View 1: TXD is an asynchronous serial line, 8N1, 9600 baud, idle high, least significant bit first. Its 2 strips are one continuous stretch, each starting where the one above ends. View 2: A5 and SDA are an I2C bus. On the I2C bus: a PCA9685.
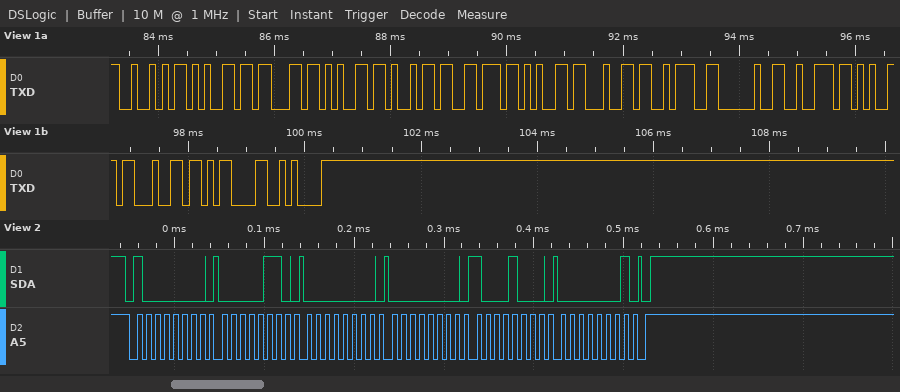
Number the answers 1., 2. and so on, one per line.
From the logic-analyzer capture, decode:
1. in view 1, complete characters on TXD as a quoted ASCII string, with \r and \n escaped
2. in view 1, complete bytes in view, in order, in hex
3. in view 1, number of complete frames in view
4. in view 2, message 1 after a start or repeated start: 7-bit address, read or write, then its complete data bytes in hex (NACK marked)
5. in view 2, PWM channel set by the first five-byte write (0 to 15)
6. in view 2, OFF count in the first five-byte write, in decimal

1. "Received: red\r\n"
2. 52 65 63 65 69 76 65 64 3A 20 72 65 64 0D 0A
3. 15
4. 0x40 write: 06 00 00 88 01
5. 0
6. 392
